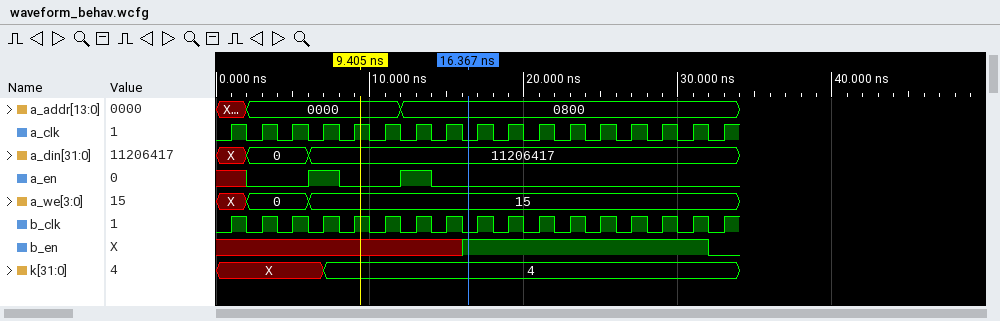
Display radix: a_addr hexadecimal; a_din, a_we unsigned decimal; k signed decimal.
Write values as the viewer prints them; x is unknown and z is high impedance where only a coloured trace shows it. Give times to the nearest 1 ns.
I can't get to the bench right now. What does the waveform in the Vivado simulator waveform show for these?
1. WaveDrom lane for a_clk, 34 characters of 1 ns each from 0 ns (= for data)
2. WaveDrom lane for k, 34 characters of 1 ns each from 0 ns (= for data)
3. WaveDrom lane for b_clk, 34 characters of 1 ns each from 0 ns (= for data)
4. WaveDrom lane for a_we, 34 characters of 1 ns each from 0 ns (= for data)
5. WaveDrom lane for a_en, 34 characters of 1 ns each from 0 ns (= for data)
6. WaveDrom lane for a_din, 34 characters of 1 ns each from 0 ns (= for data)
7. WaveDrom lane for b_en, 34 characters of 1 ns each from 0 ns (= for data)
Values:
{name: 'a_clk', wave: '0101010101010101010101010101010101'}
{name: 'k', wave: 'x......=..........................', data: '4'}
{name: 'b_clk', wave: '0101010101010101010101010101010101'}
{name: 'a_we', wave: 'x.=...=...........................', data: '0 15'}
{name: 'a_en', wave: 'x.0...1.0...1.0...................'}
{name: 'a_din', wave: 'x.=...=...........................', data: '0 11206417'}
{name: 'b_en', wave: 'x...............1...............0.'}
